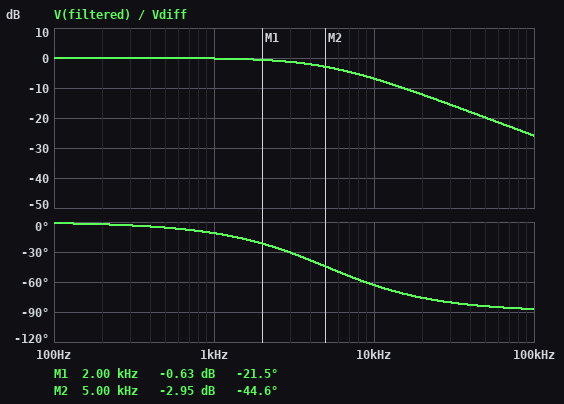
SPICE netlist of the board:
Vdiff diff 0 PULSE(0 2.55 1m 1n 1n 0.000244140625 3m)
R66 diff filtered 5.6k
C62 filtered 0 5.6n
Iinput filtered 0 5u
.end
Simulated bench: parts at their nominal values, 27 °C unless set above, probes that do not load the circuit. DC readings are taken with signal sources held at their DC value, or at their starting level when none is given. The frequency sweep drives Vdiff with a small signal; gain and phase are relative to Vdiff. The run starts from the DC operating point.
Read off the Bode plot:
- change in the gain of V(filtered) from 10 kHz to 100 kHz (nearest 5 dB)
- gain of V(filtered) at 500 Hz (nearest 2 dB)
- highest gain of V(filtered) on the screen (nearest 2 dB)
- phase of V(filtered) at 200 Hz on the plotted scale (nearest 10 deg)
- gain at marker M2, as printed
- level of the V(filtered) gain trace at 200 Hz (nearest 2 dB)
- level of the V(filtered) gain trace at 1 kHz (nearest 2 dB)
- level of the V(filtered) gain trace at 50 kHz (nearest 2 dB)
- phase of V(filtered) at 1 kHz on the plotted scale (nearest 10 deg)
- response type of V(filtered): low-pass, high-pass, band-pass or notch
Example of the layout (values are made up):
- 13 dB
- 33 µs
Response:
- -20 dB
- 0 dB
- 0 dB
- 0 deg
- -2.95 dB
- 0 dB
- 0 dB
- -20 dB
- -10 deg
- low-pass
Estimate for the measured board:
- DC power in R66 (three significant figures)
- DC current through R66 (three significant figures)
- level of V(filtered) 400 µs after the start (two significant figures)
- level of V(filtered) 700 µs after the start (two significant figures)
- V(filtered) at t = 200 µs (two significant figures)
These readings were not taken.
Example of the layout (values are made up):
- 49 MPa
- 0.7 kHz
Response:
- 140 nW
- 5.00 µA
- -28 mV
- -28 mV
- -28 mV
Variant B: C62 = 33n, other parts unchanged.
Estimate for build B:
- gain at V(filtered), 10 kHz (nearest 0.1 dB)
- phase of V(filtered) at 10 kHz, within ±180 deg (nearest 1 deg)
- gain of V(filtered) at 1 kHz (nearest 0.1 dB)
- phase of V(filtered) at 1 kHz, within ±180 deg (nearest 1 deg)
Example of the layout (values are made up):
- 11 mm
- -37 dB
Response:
- -21.3 dB
- -85 deg
- -3.7 dB
- -49 deg
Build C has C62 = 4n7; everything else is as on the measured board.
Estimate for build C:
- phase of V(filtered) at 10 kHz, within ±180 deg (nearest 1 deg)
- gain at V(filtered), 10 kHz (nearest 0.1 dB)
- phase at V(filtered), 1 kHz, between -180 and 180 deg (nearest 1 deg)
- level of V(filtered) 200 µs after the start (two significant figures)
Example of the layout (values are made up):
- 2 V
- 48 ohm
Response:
- -59 deg
- -5.7 dB
- -9 deg
- -28 mV
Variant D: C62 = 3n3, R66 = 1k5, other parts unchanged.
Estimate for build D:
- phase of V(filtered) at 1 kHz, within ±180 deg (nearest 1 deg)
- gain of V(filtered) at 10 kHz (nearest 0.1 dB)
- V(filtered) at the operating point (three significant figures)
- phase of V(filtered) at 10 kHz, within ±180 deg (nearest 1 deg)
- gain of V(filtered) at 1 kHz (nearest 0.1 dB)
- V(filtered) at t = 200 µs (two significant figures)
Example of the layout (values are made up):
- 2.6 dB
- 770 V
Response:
- -2 deg
- -0.4 dB
- -7.50 mV
- -17 deg
- 0 dB
- -7.5 mV
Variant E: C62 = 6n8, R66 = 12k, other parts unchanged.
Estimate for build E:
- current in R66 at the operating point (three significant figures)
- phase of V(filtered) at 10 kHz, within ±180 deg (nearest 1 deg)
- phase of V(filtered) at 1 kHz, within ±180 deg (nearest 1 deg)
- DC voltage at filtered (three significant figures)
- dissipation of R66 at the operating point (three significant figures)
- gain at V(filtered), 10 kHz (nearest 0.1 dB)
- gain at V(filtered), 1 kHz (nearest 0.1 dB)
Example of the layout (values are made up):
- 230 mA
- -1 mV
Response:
- 5.00 µA
- -79 deg
- -27 deg
- -60.0 mV
- 300 nW
- -14.4 dB
- -1.0 dB
